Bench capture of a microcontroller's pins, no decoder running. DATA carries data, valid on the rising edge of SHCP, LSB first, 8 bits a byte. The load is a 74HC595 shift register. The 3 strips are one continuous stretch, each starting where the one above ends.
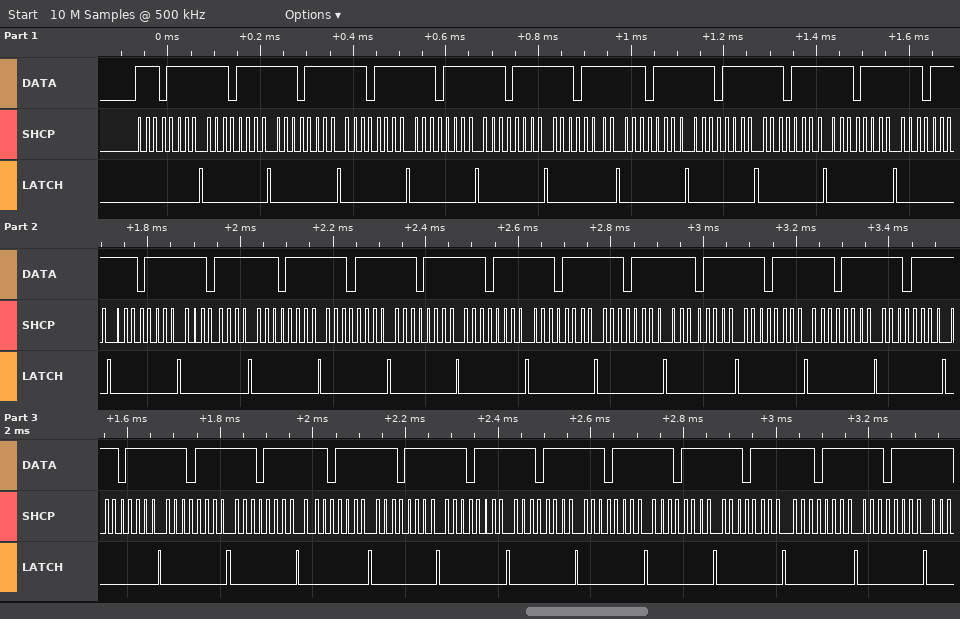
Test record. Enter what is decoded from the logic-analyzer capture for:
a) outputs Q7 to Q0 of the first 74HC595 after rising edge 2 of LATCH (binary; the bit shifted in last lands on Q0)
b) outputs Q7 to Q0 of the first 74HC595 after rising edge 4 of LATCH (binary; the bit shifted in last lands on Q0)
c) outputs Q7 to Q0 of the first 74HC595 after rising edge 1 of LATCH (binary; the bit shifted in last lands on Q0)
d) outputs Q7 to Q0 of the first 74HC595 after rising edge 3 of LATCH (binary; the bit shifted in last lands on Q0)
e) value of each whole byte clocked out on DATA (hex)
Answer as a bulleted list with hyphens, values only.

- 11101111
- 11101111
- 11101111
- 11101111
- 0xF7 0xF7 0xF7 0xF7 0xF7 0xF7 0xF7 0xF7 0xF7 0xF7 0xF7 0xF7 0xF7 0xF7 0xF7 0xF7 0xF7 0xF7 0xF7 0xF7 0xF7 0xF7 0xF7 0xF7 0xF7 0xF7 0xF7 0xF7 0xF7 0xF7 0xF7 0xF7 0xF7 0xF7 0xF7 0xF7
